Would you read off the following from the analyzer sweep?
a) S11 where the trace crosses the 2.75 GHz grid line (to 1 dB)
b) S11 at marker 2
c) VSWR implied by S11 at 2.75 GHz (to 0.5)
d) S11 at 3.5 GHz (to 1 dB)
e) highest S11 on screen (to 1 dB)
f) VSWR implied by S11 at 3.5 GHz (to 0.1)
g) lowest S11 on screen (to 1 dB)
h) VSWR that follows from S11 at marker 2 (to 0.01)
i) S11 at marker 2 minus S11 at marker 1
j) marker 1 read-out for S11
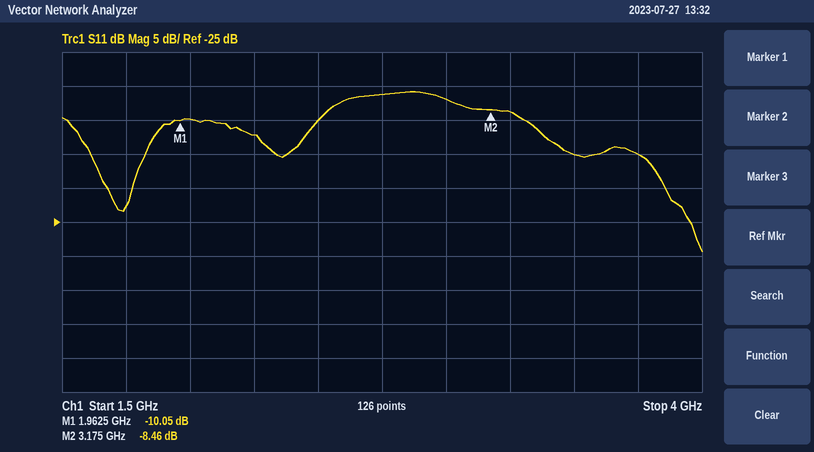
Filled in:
-6 dB
-8.46 dB
3.0
-15 dB
-6 dB
1.4
-29 dB
2.21
1.59 dB
-10.05 dB
